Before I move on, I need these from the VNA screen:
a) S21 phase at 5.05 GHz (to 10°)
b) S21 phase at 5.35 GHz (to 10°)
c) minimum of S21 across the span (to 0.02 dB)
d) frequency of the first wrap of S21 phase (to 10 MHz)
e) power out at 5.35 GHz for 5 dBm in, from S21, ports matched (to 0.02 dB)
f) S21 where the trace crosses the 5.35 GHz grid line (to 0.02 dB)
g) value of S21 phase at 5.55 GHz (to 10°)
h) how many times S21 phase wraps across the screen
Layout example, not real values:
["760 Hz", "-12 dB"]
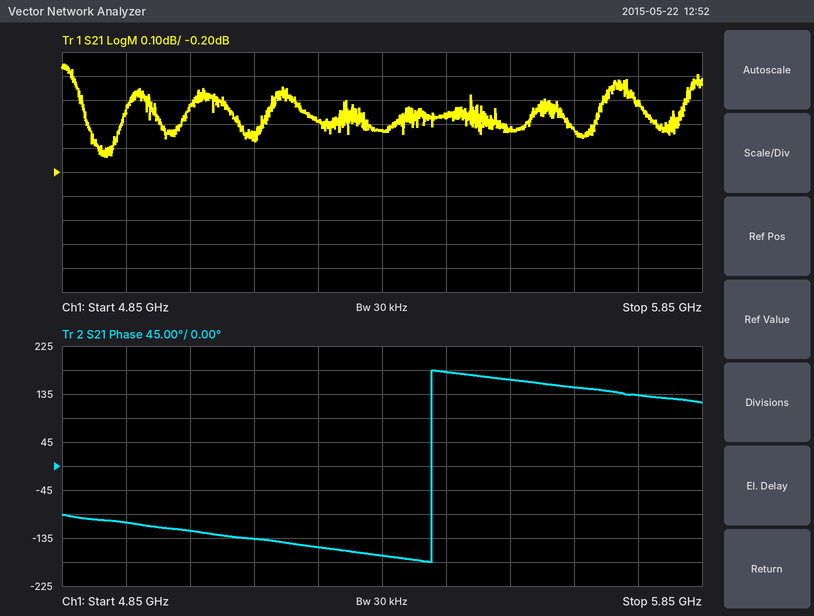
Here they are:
["-120°", "-170°", "-0.14 dB", "5.43 GHz", "4.98 dBm", "-0.02 dB", "160°", "1"]
